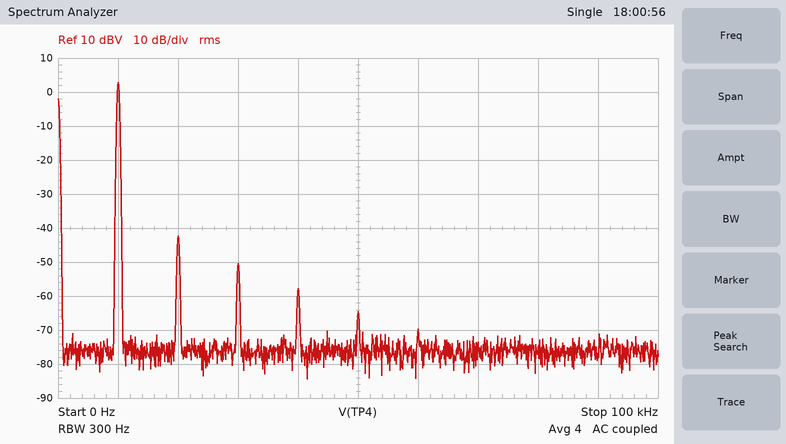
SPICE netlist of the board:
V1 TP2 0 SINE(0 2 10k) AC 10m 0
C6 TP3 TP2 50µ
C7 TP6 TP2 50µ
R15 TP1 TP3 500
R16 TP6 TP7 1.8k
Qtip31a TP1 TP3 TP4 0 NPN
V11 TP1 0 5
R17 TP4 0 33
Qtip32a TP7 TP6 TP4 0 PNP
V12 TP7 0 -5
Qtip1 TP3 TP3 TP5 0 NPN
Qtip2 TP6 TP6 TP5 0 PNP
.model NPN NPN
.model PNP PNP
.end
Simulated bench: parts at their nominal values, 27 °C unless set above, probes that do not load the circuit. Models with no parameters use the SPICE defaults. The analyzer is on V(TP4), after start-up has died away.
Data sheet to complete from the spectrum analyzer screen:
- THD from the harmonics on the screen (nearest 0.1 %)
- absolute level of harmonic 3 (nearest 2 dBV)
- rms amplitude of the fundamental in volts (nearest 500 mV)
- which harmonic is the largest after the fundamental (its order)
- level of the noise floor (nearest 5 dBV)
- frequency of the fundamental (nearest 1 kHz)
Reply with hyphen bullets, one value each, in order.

- 0.6 %
- -50 dBV
- 1.5 V
- 2
- -75 dBV
- 10 kHz
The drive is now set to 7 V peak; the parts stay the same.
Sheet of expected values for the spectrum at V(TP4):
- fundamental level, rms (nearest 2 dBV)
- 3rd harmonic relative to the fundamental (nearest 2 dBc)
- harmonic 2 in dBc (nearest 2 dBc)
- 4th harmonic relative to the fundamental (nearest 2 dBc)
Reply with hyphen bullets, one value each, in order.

- 10 dBV
- -16 dBc
- -56 dBc
- -56 dBc
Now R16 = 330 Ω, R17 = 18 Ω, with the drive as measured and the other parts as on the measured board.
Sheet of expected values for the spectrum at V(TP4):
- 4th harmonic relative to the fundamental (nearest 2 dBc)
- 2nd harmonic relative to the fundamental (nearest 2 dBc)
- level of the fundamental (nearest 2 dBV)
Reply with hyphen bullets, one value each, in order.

- -52 dBc
- -44 dBc
- 2 dBV
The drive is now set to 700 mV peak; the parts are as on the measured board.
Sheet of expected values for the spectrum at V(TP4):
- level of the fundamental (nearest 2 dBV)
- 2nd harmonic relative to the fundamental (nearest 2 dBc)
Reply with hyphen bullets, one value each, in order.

- -6 dBV
- -60 dBc
